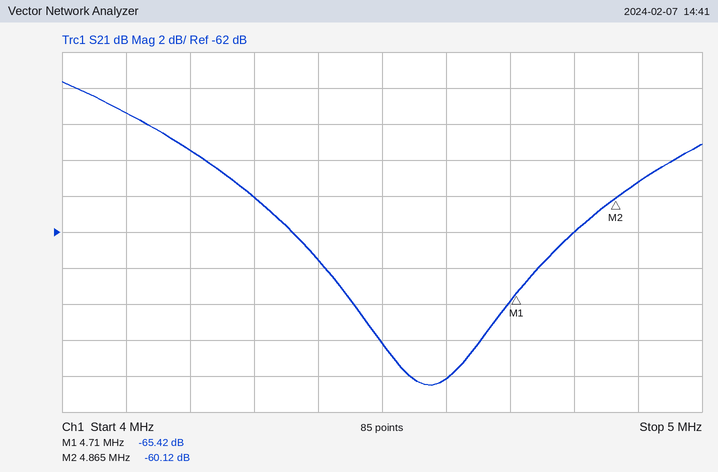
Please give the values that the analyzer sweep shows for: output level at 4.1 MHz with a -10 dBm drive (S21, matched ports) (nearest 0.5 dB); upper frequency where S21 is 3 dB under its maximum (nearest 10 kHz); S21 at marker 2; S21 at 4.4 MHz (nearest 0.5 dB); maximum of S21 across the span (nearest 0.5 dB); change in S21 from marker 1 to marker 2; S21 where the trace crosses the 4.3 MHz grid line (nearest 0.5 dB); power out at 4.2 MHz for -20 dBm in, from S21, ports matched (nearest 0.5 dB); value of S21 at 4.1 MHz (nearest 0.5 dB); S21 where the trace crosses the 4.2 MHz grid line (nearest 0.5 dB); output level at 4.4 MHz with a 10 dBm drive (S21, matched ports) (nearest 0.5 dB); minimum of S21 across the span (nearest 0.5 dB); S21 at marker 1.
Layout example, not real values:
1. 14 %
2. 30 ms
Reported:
1. -65.5 dBm
2. 4.16 MHz
3. -60.12 dB
4. -63.5 dB
5. -53.5 dB
6. 5.30 dB
7. -60.0 dB
8. -77.5 dBm
9. -55.5 dB
10. -57.5 dB
11. -53.5 dBm
12. -70.5 dB
13. -65.42 dB
